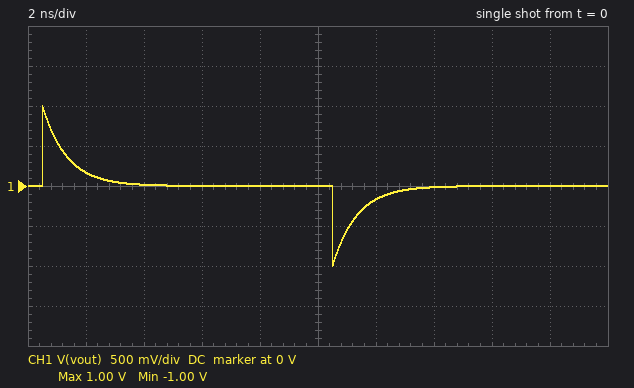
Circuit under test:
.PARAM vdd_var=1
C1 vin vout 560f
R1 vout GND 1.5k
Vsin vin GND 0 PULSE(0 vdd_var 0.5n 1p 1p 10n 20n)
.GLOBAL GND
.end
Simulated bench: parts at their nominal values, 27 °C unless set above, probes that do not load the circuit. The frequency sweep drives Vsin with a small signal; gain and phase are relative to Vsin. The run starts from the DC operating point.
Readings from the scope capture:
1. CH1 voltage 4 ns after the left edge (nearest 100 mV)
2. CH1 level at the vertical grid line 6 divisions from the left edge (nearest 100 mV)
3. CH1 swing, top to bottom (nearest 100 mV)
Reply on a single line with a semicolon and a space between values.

0 V; -200 mV; 2.0 V
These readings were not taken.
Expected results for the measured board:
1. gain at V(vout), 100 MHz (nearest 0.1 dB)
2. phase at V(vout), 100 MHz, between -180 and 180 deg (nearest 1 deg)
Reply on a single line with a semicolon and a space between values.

-6.6 dB; 62 deg
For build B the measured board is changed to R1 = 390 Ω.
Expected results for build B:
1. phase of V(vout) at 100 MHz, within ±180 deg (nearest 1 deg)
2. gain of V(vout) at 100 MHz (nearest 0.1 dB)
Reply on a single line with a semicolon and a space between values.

82 deg; -17.3 dB
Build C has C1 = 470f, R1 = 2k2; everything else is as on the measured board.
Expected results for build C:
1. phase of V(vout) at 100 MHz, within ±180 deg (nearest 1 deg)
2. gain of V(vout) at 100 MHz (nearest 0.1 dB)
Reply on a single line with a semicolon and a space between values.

57 deg; -5.3 dB
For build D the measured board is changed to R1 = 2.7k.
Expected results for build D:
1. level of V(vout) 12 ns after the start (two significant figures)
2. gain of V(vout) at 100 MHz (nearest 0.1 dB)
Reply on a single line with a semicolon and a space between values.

-370 mV; -3.2 dB
